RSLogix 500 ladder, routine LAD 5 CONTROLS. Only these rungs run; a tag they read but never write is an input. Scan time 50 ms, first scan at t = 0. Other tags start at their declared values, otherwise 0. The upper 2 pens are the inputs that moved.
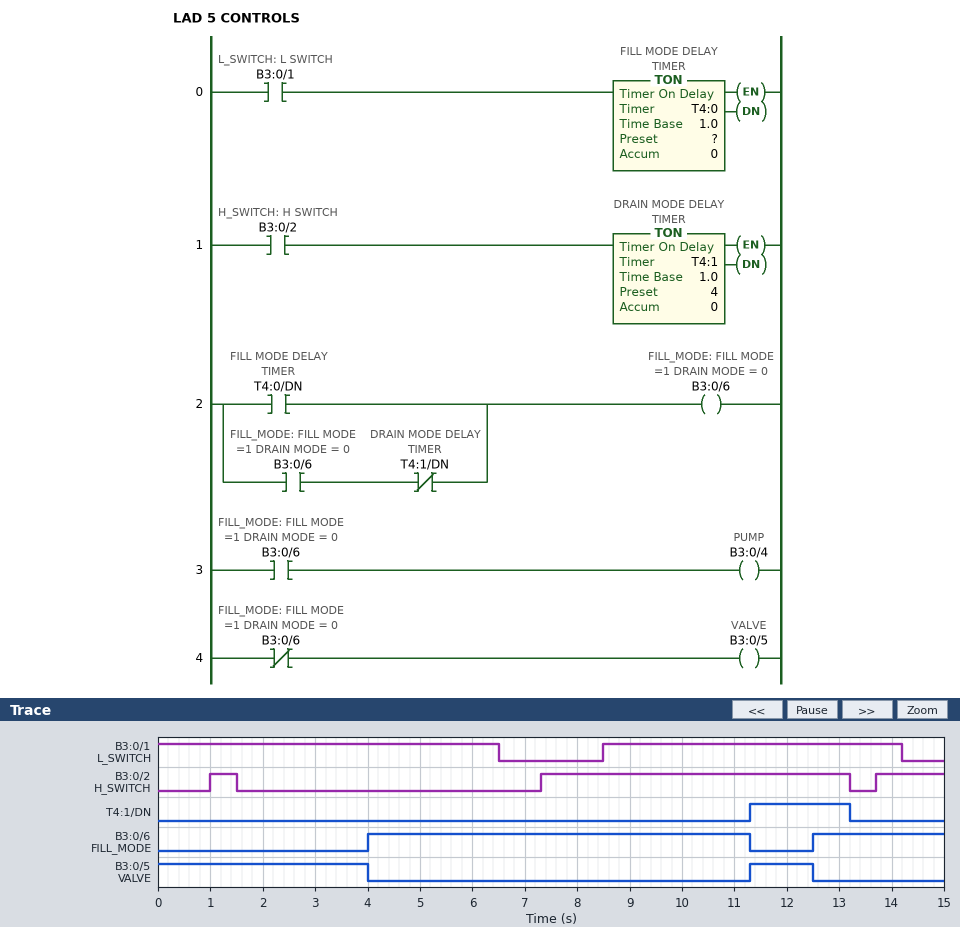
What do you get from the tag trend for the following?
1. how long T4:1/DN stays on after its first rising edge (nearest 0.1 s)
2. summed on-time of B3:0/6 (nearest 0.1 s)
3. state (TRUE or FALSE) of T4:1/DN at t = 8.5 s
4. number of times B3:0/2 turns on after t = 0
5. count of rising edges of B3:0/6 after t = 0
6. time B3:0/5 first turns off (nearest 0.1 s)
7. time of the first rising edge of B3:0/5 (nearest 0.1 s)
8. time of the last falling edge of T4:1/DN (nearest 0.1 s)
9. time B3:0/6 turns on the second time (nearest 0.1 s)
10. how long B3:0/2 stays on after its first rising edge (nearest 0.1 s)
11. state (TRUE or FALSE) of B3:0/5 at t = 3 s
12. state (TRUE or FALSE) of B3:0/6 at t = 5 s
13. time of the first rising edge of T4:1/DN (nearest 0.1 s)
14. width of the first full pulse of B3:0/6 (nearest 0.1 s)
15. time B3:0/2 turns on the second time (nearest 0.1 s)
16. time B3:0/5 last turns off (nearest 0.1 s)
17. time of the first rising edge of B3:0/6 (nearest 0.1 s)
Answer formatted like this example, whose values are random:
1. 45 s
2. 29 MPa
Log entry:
1. 1.9 s
2. 9.8 s
3. FALSE
4. 3
5. 2
6. 4.0 s
7. 11.3 s
8. 13.2 s
9. 12.5 s
10. 0.5 s
11. TRUE
12. TRUE
13. 11.3 s
14. 7.3 s
15. 7.3 s
16. 12.5 s
17. 4.0 s
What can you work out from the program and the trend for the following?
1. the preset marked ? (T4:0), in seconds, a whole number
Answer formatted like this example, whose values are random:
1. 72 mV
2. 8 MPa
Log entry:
1. 4 s
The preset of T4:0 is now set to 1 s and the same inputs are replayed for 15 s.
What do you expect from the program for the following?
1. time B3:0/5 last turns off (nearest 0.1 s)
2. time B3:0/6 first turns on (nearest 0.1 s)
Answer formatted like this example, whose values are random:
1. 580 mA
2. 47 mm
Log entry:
1. 1.0 s
2. 1.0 s
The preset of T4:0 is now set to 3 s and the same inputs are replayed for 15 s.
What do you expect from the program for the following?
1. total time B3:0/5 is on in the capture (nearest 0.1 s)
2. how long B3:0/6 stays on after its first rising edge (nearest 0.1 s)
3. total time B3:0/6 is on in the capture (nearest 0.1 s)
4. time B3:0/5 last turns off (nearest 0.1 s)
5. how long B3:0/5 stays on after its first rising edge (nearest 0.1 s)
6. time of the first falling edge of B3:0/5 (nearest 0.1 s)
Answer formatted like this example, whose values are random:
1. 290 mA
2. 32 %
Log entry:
1. 3.2 s
2. 8.3 s
3. 11.8 s
4. 11.5 s
5. 0.2 s
6. 3.0 s
